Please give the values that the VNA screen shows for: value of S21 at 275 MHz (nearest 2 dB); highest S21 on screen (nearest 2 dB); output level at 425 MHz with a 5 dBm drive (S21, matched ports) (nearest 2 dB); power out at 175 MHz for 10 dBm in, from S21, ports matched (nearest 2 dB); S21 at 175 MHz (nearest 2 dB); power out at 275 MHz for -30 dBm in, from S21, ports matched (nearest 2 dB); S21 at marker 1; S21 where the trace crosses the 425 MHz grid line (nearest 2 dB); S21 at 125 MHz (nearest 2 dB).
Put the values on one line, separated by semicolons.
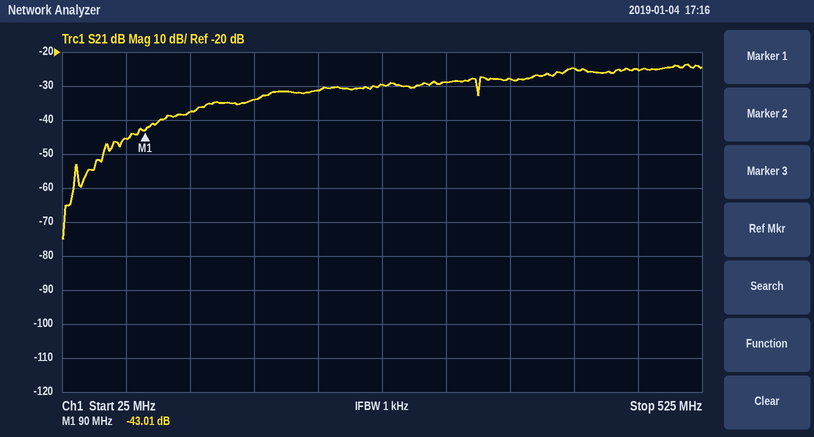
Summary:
-30 dB; -24 dB; -20 dBm; -24 dBm; -34 dB; -60 dBm; -43.01 dB; -24 dB; -38 dB
